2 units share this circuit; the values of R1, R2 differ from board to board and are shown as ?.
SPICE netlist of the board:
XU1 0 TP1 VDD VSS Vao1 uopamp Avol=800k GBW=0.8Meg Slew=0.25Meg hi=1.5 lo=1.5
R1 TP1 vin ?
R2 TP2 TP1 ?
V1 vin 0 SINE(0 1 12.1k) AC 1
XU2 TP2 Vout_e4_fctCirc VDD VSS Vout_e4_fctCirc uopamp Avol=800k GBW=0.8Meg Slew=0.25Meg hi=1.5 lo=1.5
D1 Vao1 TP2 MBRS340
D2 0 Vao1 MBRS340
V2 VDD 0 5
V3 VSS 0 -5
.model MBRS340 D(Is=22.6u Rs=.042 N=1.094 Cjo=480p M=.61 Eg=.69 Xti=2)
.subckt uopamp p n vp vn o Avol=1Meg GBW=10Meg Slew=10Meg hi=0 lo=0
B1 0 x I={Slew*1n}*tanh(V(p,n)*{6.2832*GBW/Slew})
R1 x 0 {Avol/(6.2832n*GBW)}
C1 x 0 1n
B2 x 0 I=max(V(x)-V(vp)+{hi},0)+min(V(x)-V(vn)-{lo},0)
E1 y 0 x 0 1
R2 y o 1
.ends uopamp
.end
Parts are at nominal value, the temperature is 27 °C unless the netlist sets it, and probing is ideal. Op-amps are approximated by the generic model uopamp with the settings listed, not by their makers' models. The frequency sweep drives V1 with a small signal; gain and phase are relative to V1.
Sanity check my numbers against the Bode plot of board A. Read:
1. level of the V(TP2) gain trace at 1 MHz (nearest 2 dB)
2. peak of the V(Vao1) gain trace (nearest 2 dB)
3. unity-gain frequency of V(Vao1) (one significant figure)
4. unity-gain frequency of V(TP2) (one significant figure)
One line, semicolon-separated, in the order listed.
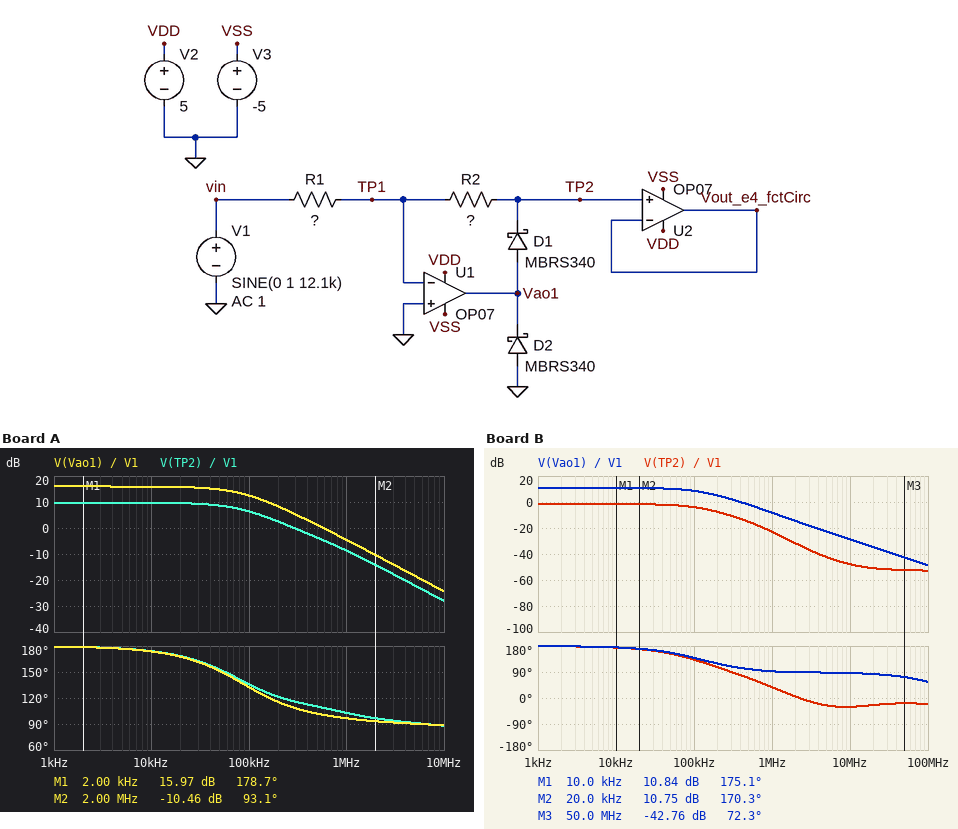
-8 dB; 16 dB; 600 kHz; 300 kHz
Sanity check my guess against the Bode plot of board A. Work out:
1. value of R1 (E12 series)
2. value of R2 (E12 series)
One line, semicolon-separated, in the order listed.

390 Ω; 1.2 kΩ
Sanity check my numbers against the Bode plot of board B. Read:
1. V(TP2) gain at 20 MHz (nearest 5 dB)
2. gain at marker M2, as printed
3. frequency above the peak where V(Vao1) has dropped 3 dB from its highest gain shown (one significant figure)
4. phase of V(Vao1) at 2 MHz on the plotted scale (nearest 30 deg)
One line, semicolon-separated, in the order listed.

-50 dB; 10.75 dB; 100 kHz; 90 deg
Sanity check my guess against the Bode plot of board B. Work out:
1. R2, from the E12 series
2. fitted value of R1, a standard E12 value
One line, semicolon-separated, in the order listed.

390 Ω; 470 Ω
